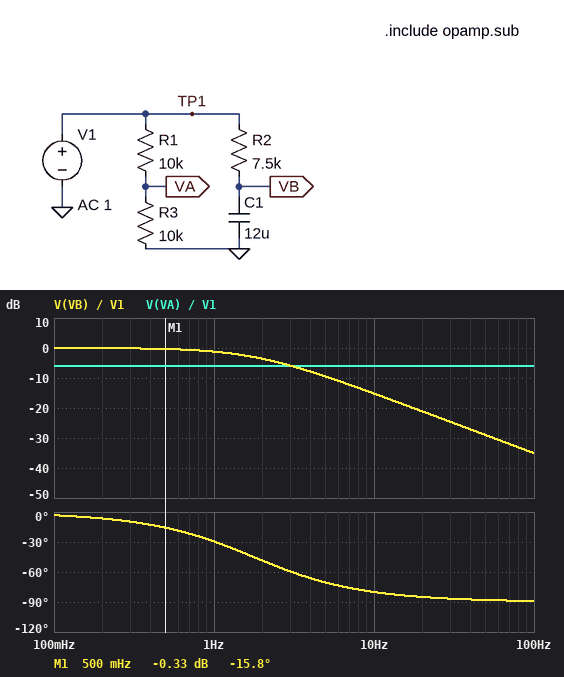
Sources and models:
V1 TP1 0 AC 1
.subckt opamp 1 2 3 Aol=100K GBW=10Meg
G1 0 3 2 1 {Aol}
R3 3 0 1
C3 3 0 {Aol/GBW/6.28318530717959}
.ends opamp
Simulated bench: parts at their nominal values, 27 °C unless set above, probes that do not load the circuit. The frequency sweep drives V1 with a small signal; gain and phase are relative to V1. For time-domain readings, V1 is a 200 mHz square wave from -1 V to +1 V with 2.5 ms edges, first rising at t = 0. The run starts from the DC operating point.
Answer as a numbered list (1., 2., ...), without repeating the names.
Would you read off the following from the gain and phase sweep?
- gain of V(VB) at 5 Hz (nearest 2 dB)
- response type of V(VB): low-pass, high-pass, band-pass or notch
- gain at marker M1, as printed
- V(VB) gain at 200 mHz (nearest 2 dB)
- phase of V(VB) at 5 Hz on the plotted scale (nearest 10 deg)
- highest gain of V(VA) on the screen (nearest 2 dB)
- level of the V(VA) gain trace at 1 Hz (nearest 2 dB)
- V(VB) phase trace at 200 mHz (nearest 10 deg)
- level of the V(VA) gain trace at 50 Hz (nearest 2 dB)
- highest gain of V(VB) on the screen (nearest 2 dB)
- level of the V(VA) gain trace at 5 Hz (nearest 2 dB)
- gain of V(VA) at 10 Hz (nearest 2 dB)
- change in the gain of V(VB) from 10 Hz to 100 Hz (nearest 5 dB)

1. -10 dB
2. low-pass
3. -0.33 dB
4. 0 dB
5. -70 deg
6. -6 dB
7. -6 dB
8. -10 deg
9. -6 dB
10. 0 dB
11. -6 dB
12. -6 dB
13. -20 dB
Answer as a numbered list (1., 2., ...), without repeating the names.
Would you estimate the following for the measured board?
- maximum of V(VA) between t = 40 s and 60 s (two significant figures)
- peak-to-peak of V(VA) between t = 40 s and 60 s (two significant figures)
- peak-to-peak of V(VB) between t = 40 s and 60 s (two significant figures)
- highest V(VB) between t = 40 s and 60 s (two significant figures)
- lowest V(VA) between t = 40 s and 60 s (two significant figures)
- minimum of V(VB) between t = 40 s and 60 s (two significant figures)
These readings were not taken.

1. 500 mV
2. 1.0 V
3. 2.0 V
4. 1.0 V
5. -500 mV
6. -1.0 V
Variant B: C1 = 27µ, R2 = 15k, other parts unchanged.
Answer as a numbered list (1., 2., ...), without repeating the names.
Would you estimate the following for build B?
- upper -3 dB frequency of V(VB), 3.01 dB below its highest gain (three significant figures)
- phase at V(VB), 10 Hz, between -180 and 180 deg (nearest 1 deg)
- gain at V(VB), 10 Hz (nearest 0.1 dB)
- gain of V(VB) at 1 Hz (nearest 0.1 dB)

1. 393 mHz
2. -88 deg
3. -28.1 dB
4. -8.7 dB
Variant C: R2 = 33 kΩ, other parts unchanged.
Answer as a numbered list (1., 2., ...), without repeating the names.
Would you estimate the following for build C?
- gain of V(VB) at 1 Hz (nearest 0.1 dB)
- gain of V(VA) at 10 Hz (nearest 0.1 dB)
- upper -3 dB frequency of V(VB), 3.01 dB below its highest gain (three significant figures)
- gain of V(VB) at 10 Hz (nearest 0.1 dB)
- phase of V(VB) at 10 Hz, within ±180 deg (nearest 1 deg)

1. -8.6 dB
2. -6.0 dB
3. 402 mHz
4. -27.9 dB
5. -88 deg
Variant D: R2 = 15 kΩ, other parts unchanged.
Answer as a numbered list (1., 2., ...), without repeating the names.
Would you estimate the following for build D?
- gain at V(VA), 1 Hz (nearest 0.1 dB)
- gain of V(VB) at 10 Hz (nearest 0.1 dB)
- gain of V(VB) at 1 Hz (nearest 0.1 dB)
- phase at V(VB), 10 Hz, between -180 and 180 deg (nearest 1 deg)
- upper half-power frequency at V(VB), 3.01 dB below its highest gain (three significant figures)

1. -6.0 dB
2. -21.1 dB
3. -3.6 dB
4. -85 deg
5. 884 mHz
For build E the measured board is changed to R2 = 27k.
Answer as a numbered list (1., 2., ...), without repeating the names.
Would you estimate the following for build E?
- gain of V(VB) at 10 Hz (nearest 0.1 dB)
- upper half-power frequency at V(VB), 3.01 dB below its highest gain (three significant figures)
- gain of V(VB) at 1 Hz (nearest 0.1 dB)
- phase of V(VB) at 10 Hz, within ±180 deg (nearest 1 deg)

1. -26.2 dB
2. 491 mHz
3. -7.1 dB
4. -87 deg
